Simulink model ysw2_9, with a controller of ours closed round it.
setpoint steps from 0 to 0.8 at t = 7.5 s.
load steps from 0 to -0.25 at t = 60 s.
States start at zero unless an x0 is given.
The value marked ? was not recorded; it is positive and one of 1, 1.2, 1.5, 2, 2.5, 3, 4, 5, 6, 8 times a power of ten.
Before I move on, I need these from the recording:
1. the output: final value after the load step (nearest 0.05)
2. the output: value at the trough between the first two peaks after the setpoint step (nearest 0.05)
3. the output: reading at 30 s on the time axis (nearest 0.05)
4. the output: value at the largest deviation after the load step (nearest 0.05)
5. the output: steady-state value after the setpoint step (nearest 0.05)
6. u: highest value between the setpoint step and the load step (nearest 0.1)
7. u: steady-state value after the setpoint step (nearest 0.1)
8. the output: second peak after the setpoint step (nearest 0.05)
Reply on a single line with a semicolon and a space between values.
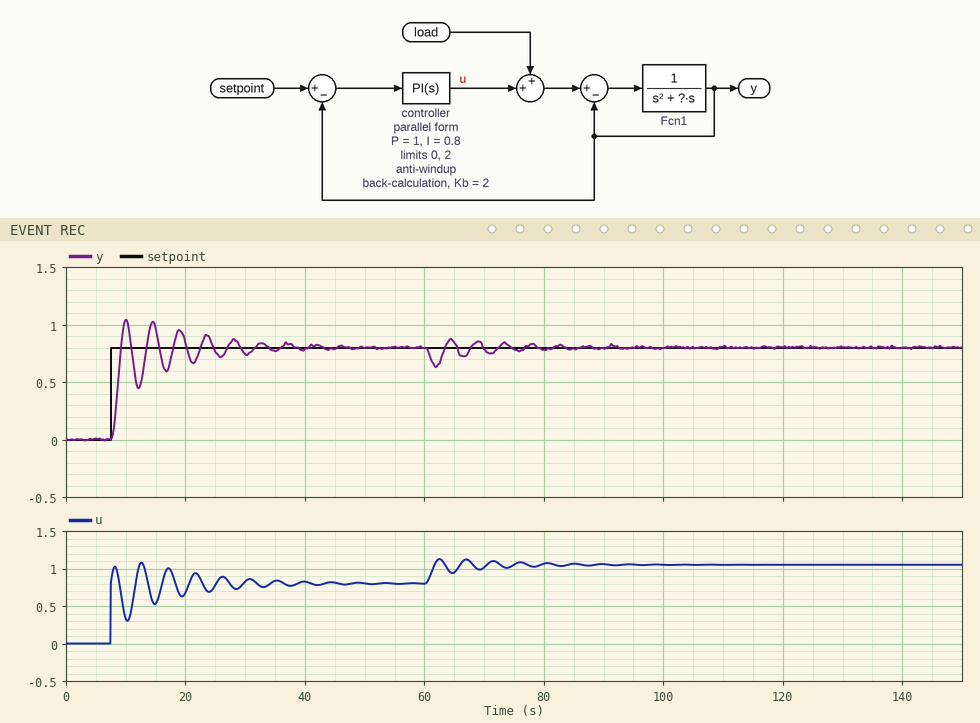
0.80; 0.45; 0.75; 0.65; 0.80; 1.1; 0.8; 1.00
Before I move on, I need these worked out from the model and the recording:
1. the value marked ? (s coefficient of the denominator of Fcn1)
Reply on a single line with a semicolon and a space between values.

0.6
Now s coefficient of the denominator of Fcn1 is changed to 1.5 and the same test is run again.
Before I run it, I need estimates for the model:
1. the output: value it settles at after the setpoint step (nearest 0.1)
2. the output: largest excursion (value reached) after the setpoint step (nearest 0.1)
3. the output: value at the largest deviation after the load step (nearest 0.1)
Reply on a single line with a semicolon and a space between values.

0.8; 0.9; 0.7
